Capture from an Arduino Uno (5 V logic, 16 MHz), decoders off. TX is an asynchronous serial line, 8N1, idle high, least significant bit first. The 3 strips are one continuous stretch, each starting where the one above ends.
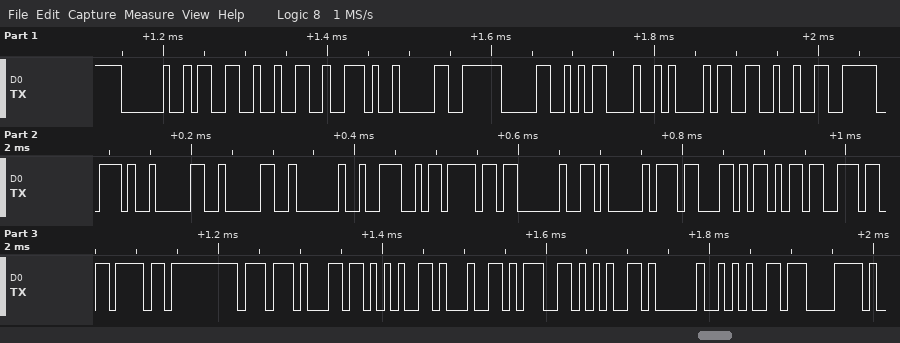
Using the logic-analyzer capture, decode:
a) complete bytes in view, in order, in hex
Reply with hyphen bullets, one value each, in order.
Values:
- 0x20 0x33 0x32 0x2E 0x30 0x30 0x0D 0x0A 0x33 0x32 0x2E 0x30 0x30 0x20 0x4E 0x6F 0x20 0x41 0x63 0x6B 0x6E 0x6F 0x77 0x6C 0x65 0x64 0x67 0x65 0x20 0x65 0x78
